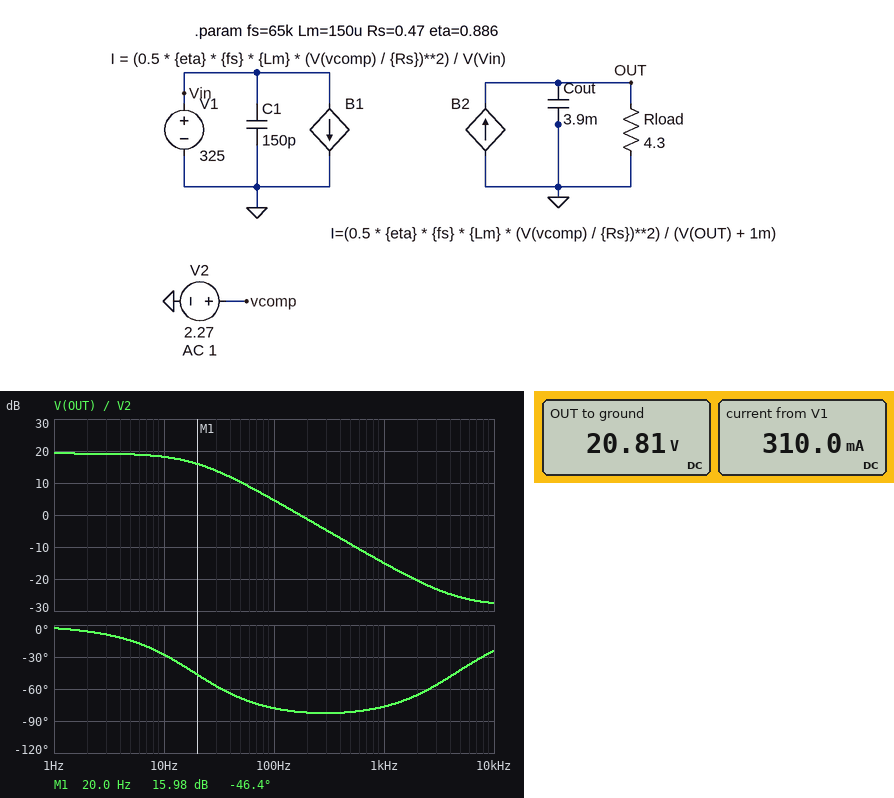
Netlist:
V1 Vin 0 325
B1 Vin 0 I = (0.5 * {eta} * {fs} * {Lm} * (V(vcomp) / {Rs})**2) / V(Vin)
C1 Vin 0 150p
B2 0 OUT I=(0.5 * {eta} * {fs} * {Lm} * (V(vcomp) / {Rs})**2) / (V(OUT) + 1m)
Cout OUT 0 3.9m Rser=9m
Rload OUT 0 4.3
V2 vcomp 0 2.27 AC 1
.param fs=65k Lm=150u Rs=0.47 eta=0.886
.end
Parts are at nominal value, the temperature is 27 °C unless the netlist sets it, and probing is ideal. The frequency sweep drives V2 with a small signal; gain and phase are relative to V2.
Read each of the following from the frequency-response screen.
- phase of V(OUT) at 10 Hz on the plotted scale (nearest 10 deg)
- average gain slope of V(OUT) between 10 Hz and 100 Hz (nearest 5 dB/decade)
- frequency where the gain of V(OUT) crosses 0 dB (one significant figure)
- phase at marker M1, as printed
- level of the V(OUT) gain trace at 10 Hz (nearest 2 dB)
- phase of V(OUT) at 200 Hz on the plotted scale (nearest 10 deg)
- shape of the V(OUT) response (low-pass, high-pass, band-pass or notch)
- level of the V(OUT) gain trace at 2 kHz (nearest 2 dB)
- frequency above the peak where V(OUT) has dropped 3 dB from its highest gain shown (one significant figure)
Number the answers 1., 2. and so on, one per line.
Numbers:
1. -30 deg
2. -15 dB/decade
3. 200 Hz
4. -46.4 deg
5. 18 dB
6. -80 deg
7. low-pass
8. -20 dB
9. 20 Hz
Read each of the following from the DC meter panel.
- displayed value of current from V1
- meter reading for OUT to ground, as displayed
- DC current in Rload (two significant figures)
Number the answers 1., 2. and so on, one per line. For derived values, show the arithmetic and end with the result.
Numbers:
1. 310.0 mA
2. 20.81 V
3. (20.81 V) / 4.3 Ω = 4.8 A
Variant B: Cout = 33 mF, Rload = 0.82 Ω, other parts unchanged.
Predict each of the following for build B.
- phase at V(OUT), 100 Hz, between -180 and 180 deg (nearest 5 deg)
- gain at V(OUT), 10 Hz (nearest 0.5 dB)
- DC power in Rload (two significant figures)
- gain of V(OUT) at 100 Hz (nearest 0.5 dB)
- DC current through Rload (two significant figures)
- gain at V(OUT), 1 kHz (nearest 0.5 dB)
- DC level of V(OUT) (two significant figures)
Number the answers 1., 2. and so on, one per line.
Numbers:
1. -75 deg
2. 9.5 dB
3. 100 W
4. -6.5 dB
5. 11 A
6. -20.0 dB
7. 9.1 V
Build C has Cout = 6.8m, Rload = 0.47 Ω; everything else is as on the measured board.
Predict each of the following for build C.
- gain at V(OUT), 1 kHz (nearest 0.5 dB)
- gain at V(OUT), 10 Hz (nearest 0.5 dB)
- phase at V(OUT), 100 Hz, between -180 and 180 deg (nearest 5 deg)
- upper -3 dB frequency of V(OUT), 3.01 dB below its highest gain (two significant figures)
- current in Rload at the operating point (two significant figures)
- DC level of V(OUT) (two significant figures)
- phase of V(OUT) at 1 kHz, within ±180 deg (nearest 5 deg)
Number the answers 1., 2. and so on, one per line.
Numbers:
1. -10.0 dB
2. 9.5 dB
3. -45 deg
4. 96 Hz
5. 15 A
6. 6.9 V
7. -65 deg
